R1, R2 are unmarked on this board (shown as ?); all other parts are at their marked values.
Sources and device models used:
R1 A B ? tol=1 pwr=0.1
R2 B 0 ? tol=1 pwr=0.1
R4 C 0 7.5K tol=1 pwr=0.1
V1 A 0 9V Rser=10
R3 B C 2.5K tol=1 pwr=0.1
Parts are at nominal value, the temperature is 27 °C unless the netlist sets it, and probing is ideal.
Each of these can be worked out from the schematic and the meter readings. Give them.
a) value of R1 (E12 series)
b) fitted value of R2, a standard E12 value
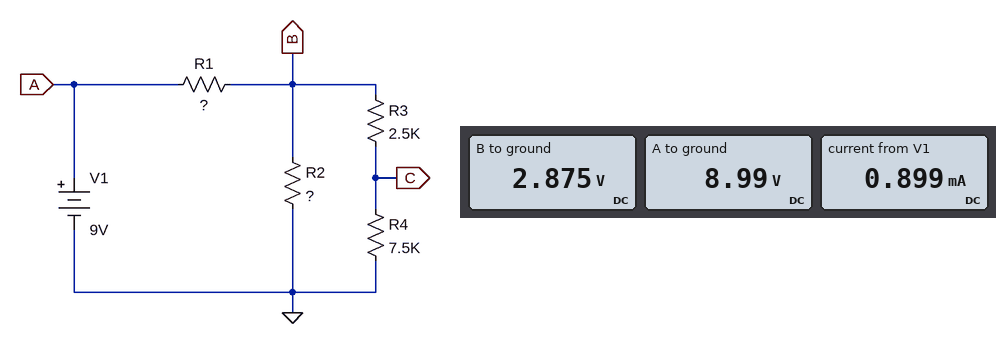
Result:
6.8 kΩ
4.7 kΩ
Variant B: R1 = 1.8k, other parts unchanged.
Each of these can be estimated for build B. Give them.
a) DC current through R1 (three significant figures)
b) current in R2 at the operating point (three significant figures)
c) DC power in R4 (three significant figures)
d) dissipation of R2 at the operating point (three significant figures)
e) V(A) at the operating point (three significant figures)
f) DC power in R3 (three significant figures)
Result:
1.80 mA
1.22 mA
2.48 mW
7.03 mW
8.98 V
826 µW
